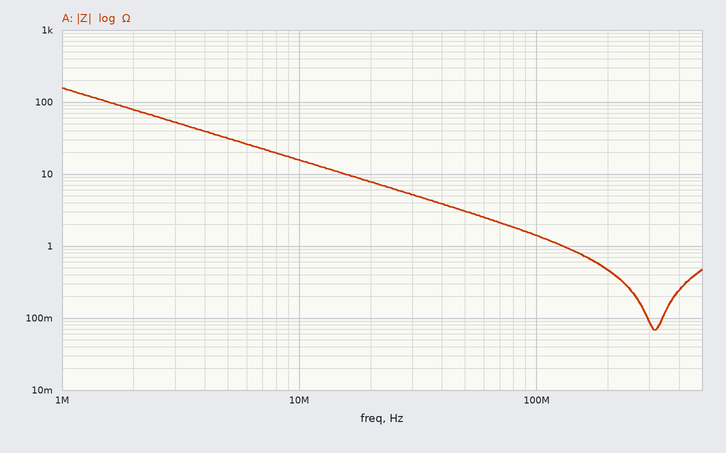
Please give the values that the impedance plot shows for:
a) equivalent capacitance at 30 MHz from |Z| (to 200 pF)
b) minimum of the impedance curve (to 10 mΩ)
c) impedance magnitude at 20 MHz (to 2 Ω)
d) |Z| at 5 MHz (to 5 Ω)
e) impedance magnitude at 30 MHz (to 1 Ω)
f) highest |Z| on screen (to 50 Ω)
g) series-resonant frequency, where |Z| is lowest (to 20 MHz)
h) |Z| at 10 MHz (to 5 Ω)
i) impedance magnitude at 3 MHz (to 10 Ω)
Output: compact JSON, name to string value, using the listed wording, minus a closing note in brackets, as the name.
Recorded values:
{"equivalent capacitance at 30 MHz from |Z|": "1.0 nF", "minimum of the impedance curve": "70 mΩ", "impedance magnitude at 20 MHz": "8 Ω", "|Z| at 5 MHz": "30 Ω", "impedance magnitude at 30 MHz": "5 Ω", "highest |Z| on screen": "150 Ω", "series-resonant frequency, where |Z| is lowest": "320 MHz", "|Z| at 10 MHz": "15 Ω", "impedance magnitude at 3 MHz": "50 Ω"}
